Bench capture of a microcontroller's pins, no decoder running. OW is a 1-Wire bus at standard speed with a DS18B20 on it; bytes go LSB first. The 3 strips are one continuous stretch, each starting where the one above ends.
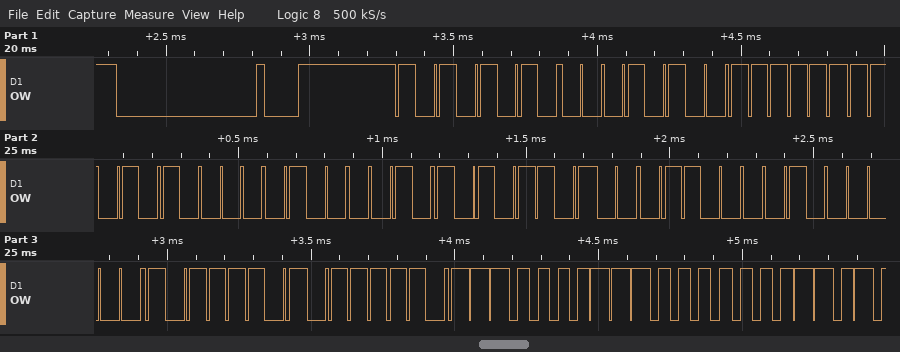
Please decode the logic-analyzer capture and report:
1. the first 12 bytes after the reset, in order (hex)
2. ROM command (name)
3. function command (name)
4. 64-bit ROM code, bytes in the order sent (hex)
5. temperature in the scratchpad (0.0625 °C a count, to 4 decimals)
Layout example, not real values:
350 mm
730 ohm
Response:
55 28 FF 0A 42 B5 18 02 BD BE C3 01
Match ROM
Read Scratchpad
28 FF 0A 42 B5 18 02 BD
28.1875 °C
